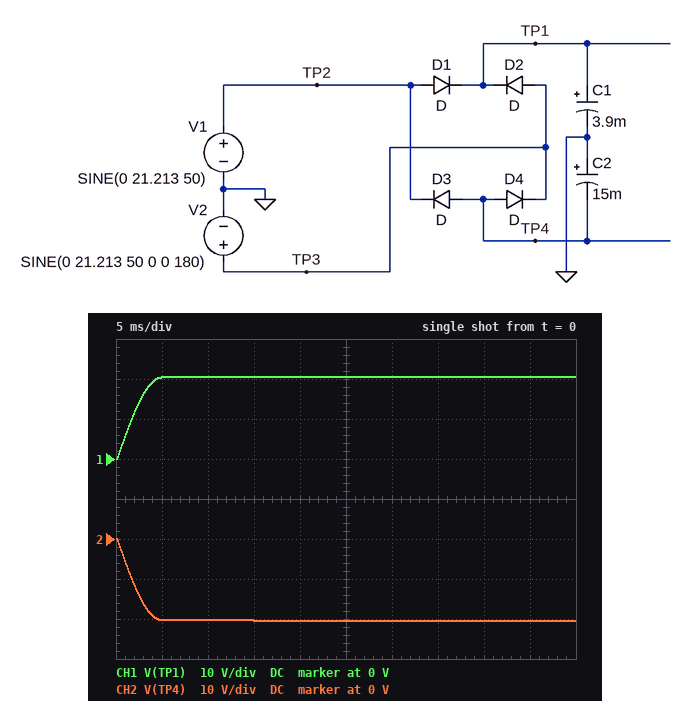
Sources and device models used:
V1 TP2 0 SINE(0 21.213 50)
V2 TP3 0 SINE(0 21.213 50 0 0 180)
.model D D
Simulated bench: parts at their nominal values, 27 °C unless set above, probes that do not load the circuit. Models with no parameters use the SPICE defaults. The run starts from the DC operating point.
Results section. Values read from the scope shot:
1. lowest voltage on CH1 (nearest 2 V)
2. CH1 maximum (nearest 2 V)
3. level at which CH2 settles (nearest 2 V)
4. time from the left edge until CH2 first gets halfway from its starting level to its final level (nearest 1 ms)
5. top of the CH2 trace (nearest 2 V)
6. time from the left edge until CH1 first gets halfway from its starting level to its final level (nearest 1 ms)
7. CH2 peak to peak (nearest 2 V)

0 V
20 V
-20 V
2 ms
0 V
2 ms
20 V
